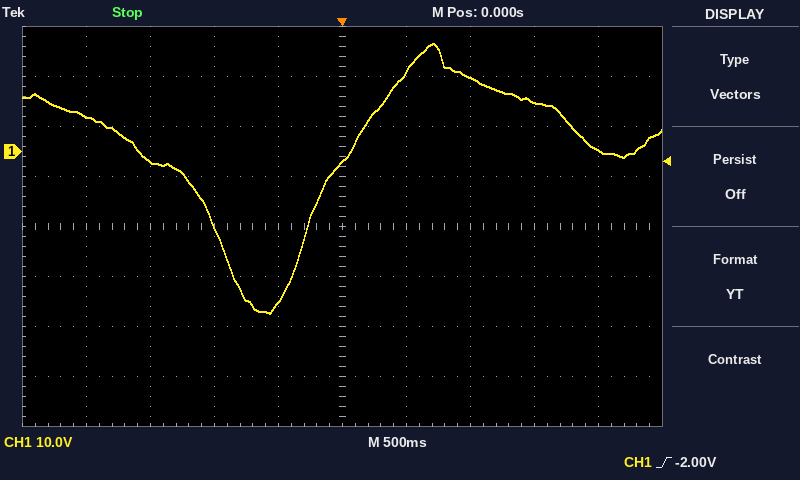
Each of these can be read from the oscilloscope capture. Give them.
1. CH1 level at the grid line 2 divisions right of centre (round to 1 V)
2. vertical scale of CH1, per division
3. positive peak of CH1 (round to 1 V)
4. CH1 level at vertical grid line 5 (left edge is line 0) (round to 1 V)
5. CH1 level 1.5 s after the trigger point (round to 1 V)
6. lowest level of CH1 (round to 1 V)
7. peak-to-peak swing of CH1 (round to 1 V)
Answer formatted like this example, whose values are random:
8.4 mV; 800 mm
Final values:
15 V; 10 V; 22 V; -2 V; 10 V; -32 V; 54 V
